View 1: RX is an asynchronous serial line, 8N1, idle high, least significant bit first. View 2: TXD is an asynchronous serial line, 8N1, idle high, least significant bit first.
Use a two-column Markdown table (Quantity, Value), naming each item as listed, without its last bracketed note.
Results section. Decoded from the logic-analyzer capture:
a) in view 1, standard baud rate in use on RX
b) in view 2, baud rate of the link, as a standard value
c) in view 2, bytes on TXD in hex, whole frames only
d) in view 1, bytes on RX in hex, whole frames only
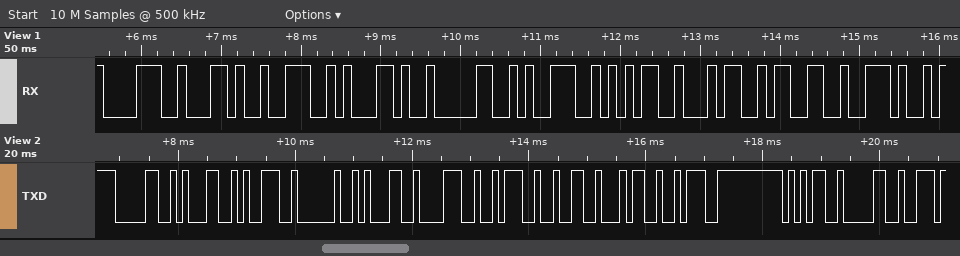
| Quantity | Value |
|---|---|
| in view 1, standard baud rate in use on RX | 9600 baud |
| in view 2, baud rate of the link, as a standard value | 9600 baud |
| in view 2, bytes on TXD in hex, whole frames only | 30 31 39 20 31 38 3A 32 34 3A 35 30 |
| in view 1, bytes on RX in hex, whole frames only | 0x38 0x2C 0x4E 0x2C 0x30 0x39 0x35 0x34 0x33 0x2E |
